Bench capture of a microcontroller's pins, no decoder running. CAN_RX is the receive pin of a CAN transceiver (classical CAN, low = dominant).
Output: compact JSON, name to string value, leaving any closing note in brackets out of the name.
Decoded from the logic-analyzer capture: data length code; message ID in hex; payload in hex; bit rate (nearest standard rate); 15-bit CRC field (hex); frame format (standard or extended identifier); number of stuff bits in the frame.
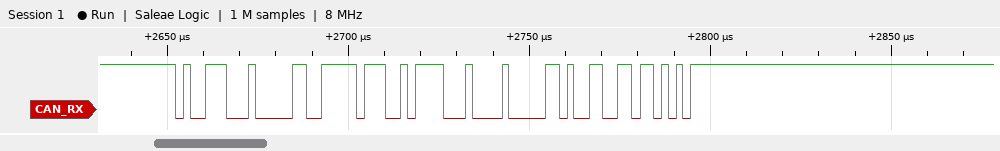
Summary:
{"data length code": "4", "message ID in hex": "0x4E2", "payload in hex": "FF 2F 10 82", "bit rate": "500 kbit/s", "15-bit CRC field": "0x4CDA", "frame format": "standard", "number of stuff bits in the frame": "3"}
